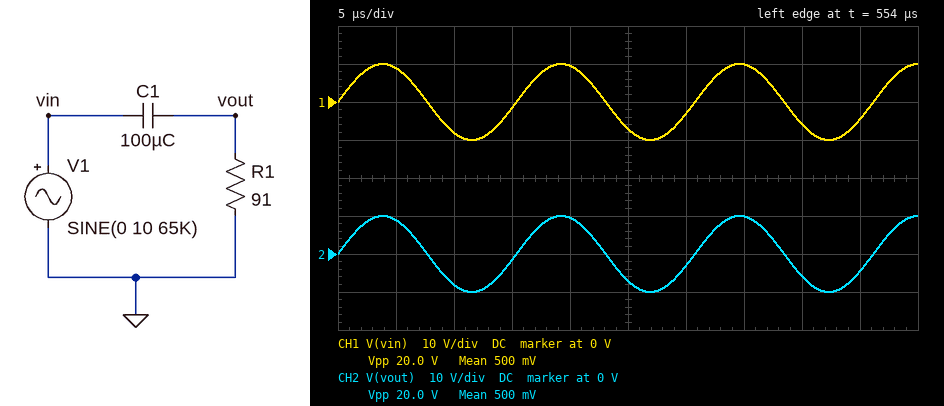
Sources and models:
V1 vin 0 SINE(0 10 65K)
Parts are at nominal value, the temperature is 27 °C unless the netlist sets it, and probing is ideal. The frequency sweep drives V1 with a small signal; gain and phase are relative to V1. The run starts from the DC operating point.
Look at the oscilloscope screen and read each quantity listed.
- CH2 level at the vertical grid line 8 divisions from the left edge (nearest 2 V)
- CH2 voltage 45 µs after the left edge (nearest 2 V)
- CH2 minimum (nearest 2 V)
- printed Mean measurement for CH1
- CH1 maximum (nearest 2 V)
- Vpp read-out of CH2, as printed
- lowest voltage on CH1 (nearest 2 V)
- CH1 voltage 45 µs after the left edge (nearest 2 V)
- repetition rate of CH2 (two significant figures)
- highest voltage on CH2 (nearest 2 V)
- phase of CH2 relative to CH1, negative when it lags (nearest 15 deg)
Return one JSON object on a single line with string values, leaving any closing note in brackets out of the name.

{"CH2 level at the vertical grid line 8 divisions from the left edge": "-6 V", "CH2 voltage 45 µs after the left edge": "-4 V", "CH2 minimum": "-10 V", "printed Mean measurement for CH1": "500 mV", "CH1 maximum": "10 V", "Vpp read-out of CH2, as printed": "20.0 V", "lowest voltage on CH1": "-10 V", "CH1 voltage 45 µs after the left edge": "-4 V", "repetition rate of CH2": "65 kHz", "highest voltage on CH2": "10 V", "phase of CH2 relative to CH1, negative when it lags": "0 deg"}
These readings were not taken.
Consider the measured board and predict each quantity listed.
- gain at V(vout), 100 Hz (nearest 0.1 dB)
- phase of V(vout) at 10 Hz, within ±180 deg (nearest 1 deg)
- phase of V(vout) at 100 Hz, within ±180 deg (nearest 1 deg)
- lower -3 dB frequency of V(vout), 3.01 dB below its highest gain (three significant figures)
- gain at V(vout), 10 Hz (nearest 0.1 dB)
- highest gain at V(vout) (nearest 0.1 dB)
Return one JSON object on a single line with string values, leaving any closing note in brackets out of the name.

{"gain at V(vout), 100 Hz": "-0.1 dB", "phase of V(vout) at 10 Hz, within ±180 deg": "60 deg", "phase of V(vout) at 100 Hz, within ±180 deg": "10 deg", "lower -3 dB frequency of V(vout), 3.01 dB below its highest gain": "17.5 Hz", "gain at V(vout), 10 Hz": "-6.1 dB", "highest gain at V(vout)": "0 dB"}
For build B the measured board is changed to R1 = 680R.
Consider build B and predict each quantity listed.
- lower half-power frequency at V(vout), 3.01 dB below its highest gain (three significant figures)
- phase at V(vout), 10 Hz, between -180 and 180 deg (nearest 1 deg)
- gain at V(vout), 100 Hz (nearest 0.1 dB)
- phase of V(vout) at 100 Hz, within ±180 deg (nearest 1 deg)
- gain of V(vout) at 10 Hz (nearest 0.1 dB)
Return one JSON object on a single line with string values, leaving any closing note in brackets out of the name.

{"lower half-power frequency at V(vout), 3.01 dB below its highest gain": "2.34 Hz", "phase at V(vout), 10 Hz, between -180 and 180 deg": "13 deg", "gain at V(vout), 100 Hz": "0 dB", "phase of V(vout) at 100 Hz, within ±180 deg": "1 deg", "gain of V(vout) at 10 Hz": "-0.2 dB"}
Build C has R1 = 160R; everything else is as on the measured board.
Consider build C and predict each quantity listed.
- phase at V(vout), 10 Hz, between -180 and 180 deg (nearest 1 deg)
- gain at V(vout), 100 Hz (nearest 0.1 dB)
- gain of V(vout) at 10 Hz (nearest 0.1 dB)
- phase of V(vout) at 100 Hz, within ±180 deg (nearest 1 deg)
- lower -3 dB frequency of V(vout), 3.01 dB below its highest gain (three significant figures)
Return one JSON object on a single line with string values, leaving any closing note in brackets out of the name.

{"phase at V(vout), 10 Hz, between -180 and 180 deg": "45 deg", "gain at V(vout), 100 Hz": "0 dB", "gain of V(vout) at 10 Hz": "-3.0 dB", "phase of V(vout) at 100 Hz, within ±180 deg": "6 deg", "lower -3 dB frequency of V(vout), 3.01 dB below its highest gain": "9.95 Hz"}
